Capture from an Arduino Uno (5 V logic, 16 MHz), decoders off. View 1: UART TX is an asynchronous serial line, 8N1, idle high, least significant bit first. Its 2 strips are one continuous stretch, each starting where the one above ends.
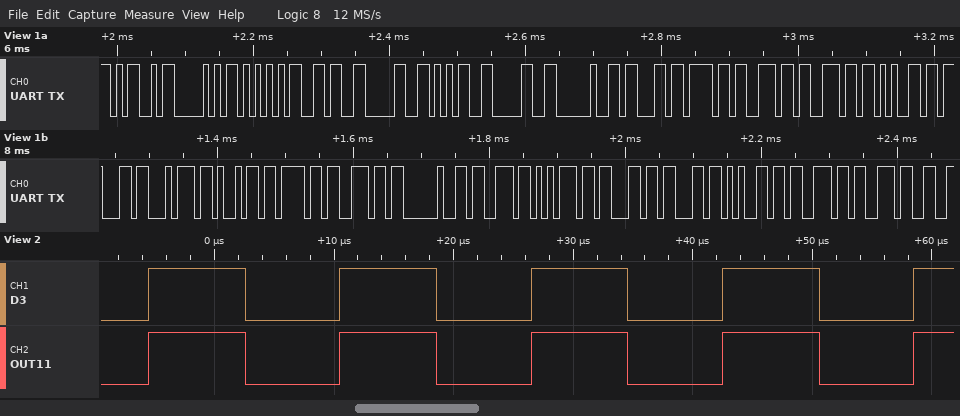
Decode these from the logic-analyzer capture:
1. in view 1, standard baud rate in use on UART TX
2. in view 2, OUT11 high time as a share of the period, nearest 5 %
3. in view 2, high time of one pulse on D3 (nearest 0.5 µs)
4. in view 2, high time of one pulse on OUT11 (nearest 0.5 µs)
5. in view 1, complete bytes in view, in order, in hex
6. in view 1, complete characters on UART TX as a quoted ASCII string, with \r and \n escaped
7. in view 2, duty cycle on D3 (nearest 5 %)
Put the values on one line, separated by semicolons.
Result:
115200 baud; 50 %; 8.0 µs; 8.0 µs; 4D 50 55 36 30 35 30 20 63 6F 6E 6E 65 63 74 69 6F 6E 20 73 75 63 63 65 73 73; "MPU6050 connection success"; 50 %
